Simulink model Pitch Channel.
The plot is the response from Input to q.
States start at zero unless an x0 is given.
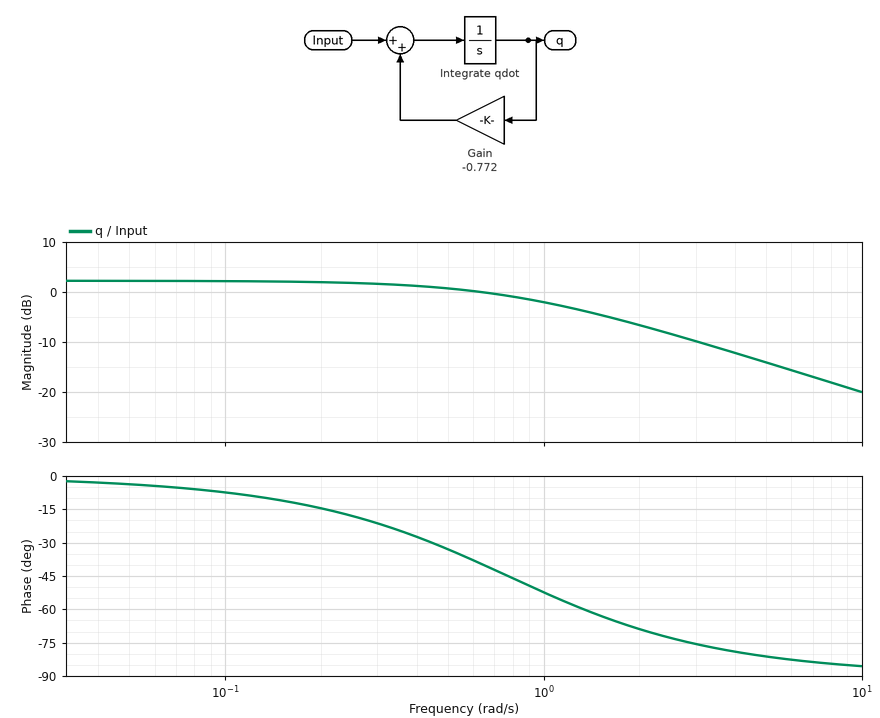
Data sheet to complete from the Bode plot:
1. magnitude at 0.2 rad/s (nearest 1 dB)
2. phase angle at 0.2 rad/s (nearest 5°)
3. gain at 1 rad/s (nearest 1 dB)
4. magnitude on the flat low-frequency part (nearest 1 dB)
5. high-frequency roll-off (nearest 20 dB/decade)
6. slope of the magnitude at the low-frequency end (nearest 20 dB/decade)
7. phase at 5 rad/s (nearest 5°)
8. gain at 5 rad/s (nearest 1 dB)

2 dB
-15°
-2 dB
2 dB
-20 dB/decade
0 dB/decade
-80°
-14 dB
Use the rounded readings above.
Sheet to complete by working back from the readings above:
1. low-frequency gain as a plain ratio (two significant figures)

1.3
